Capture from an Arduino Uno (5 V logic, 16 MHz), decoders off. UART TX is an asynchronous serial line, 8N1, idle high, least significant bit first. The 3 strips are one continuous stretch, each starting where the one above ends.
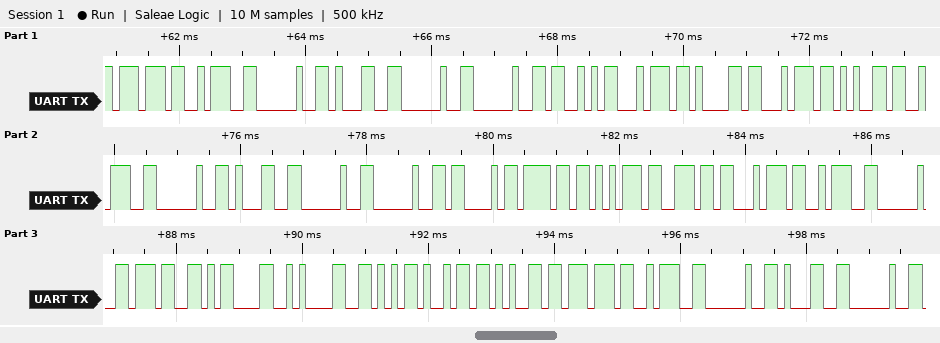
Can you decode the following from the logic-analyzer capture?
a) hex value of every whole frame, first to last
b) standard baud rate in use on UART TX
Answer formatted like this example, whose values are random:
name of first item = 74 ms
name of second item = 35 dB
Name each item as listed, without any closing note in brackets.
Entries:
hex value of every whole frame, first to last = 77 3A 20 31 20 20 53 74 61 74 65 3A 20 31 20 20 43 6F 75 6E 74 3A 20 37 0D 0A 56 69 65 77 3A 20 31 20
standard baud rate in use on UART TX = 9600 baud
